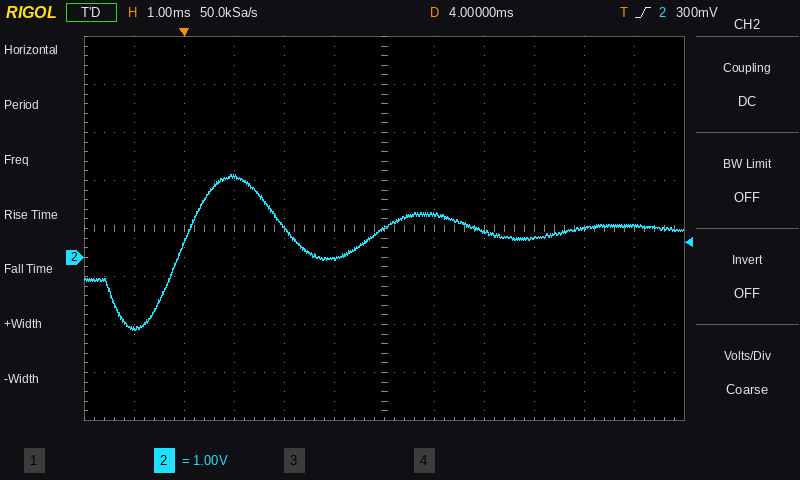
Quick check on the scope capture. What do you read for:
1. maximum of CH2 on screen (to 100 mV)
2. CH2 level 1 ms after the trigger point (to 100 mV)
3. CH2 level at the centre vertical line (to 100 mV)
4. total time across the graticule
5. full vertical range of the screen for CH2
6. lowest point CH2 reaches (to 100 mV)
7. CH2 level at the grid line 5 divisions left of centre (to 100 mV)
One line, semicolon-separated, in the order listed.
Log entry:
1.7 V; 1.7 V; 600 mV; 12 ms; 8 V; -1.5 V; -1.5 V
